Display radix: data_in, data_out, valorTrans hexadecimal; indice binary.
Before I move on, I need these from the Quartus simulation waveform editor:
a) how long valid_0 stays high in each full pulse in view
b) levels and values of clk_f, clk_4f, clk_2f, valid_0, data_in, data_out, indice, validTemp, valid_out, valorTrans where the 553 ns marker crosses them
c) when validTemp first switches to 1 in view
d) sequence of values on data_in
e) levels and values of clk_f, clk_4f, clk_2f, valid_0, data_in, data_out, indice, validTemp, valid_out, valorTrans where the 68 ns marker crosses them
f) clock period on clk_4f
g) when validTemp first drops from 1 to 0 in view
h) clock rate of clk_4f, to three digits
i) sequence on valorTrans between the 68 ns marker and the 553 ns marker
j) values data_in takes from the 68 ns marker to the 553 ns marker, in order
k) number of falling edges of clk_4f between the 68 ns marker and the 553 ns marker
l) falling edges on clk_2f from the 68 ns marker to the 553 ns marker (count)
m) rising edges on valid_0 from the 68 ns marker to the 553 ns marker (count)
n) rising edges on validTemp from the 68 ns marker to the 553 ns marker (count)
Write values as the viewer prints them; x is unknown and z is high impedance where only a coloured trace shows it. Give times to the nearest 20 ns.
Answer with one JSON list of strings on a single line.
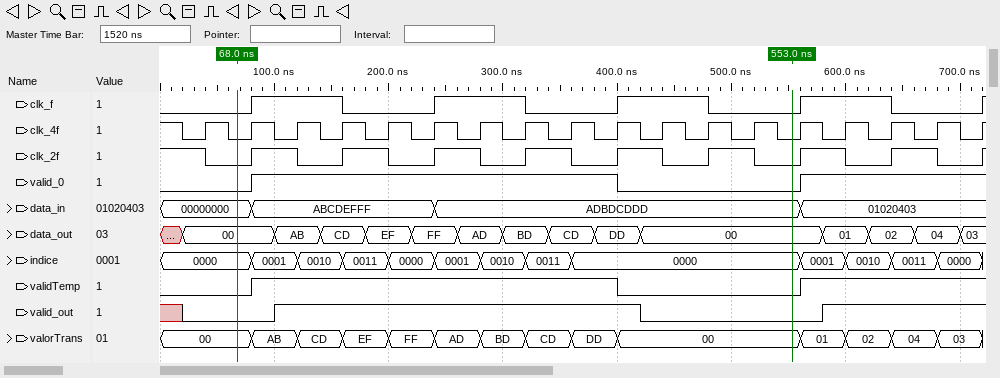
["320 ns", "clk_f=0, clk_4f=0, clk_2f=0, valid_0=0, data_in=ADBDCDDD, data_out=00, indice=0000, validTemp=0, valid_out=0, valorTrans=00", "80 ns", "00000000, ABCDEFFF, ADBDCDDD, 01020403", "clk_f=0, clk_4f=0, clk_2f=0, valid_0=0, data_in=00000000, data_out=00, indice=0000, validTemp=0, valid_out=0, valorTrans=00", "40 ns", "400 ns", "25.0 MHz", "00, AB, CD, EF, FF, AD, BD, CD, DD, 00", "00000000, ABCDEFFF, ADBDCDDD", "12", "6", "1", "1"]
